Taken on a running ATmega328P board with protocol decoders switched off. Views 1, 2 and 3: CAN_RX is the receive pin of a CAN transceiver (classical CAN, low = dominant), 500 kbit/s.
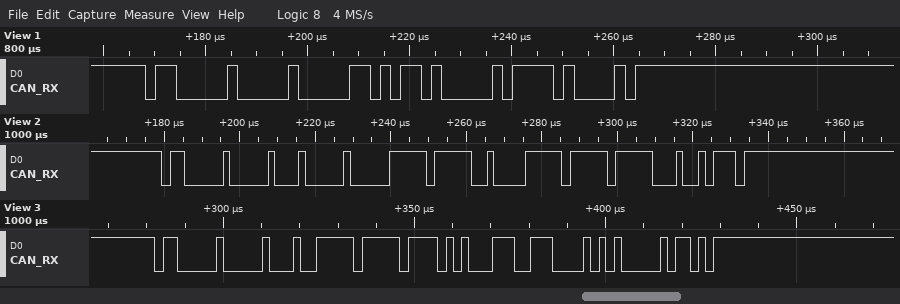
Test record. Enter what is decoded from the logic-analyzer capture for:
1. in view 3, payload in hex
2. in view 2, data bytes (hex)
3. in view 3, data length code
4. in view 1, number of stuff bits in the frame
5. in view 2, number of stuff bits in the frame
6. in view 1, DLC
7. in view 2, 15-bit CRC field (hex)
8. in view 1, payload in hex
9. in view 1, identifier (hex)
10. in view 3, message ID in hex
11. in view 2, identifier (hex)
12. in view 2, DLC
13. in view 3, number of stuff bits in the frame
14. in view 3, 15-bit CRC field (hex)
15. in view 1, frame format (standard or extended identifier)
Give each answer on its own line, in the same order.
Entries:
FF FD 47 38
00 FF A1 FF
4
4
9
1
0x7E4B
5A
0x600
0x600
0x600
4
5
0x2A06
standard
